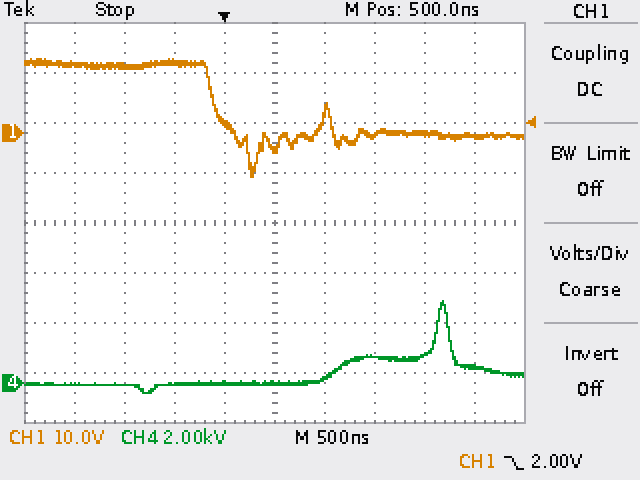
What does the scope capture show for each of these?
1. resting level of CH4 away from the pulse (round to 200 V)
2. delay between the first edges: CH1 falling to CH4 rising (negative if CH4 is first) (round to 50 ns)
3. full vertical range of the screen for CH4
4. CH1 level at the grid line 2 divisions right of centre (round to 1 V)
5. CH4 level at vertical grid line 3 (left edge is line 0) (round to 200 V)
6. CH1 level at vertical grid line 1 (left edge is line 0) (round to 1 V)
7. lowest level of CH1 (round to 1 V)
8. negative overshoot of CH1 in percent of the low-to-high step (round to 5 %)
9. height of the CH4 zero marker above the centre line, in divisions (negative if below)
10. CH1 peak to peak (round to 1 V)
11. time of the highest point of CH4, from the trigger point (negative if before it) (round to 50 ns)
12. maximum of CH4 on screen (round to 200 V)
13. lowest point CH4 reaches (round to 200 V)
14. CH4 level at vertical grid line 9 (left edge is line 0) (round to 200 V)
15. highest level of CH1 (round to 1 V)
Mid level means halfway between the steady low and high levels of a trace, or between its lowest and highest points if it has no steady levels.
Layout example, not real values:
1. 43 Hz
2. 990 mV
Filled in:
1. 0.0 kV
2. +2.20 µs
3. 16 kV
4. 0 V
5. 0.0 kV
6. 14 V
7. -9 V
8. 60 %
9. -3.2 div
10. 24 V
11. +2.20 µs
12. 3.2 kV
13. -400 V
14. 600 V
15. 15 V
